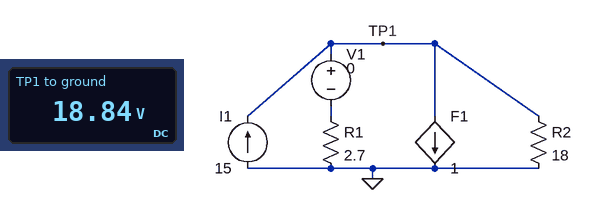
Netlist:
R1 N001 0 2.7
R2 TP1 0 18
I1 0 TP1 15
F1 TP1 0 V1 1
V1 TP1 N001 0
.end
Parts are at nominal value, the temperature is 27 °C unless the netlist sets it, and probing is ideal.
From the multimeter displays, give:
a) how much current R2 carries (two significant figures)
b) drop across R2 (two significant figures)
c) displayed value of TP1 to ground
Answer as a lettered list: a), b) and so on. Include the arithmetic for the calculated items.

a) (18.84 V) / 18 Ω = 1.0 A
b) 18.84 V = 19 V
c) 18.84 V
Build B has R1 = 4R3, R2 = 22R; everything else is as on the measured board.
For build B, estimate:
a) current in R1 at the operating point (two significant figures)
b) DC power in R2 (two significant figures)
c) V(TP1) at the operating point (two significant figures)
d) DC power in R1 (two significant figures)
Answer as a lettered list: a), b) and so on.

a) 6.8 A
b) 39 W
c) 29 V
d) 200 W
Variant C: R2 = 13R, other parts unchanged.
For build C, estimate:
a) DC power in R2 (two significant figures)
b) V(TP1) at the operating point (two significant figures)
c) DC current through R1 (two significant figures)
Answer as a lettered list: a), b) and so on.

a) 26 W
b) 18 V
c) 6.8 A
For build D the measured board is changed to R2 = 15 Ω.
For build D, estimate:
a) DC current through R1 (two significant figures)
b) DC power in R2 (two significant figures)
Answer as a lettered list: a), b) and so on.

a) 6.9 A
b) 23 W
